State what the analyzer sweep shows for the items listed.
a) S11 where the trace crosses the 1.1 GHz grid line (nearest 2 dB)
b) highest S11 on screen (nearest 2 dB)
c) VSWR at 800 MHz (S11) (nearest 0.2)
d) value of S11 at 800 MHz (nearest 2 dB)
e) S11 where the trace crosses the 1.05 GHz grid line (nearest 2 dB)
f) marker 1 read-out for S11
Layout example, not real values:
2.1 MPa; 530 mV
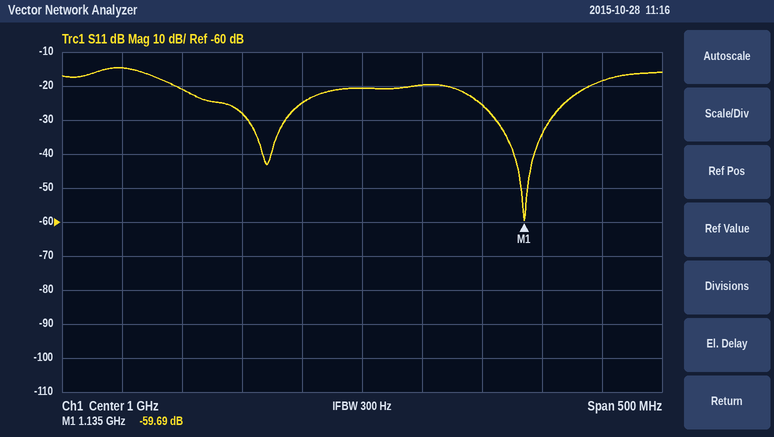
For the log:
-26 dB; -14 dB; 1.4; -14 dB; -20 dB; -59.69 dB
